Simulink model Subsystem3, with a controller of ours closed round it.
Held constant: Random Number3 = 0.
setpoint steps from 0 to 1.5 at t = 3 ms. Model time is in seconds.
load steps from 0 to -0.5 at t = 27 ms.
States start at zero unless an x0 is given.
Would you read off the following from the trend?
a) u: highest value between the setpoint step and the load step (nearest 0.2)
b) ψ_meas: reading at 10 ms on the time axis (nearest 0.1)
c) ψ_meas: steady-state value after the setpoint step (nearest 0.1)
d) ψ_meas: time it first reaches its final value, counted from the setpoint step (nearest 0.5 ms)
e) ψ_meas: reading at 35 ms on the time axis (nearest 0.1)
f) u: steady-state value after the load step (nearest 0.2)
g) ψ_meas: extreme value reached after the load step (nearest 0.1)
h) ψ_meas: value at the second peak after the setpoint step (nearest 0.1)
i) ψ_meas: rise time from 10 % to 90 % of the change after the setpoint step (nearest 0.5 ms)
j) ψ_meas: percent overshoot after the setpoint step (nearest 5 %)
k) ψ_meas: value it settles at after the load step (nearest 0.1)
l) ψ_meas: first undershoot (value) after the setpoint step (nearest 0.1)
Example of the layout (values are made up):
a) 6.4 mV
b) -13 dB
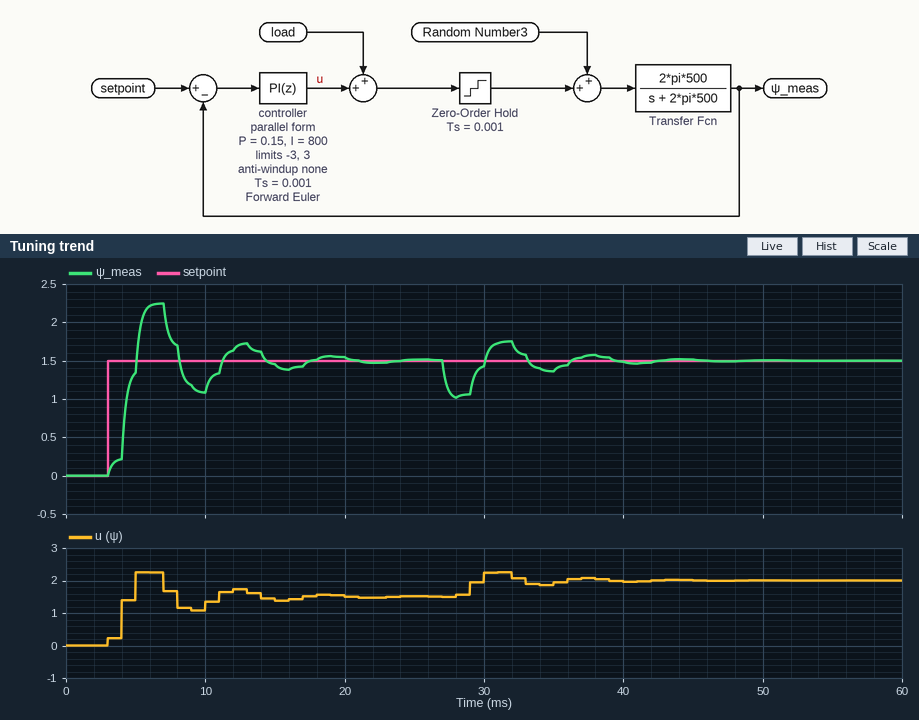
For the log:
a) 2.2
b) 1.1
c) 1.5
d) 2.0 ms
e) 1.4
f) 2.0
g) 1.0
h) 1.7
i) 1.5 ms
j) 50 %
k) 1.5
l) 1.1
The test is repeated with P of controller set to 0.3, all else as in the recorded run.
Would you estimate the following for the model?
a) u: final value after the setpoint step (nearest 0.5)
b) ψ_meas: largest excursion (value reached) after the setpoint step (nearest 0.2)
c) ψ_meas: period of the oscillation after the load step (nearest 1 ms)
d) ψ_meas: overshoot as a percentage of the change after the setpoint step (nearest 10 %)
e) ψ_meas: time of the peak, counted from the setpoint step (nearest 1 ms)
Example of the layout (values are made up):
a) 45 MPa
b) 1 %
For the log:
a) 1.5
b) 2.0
c) 6 ms
d) 40 %
e) 3 ms
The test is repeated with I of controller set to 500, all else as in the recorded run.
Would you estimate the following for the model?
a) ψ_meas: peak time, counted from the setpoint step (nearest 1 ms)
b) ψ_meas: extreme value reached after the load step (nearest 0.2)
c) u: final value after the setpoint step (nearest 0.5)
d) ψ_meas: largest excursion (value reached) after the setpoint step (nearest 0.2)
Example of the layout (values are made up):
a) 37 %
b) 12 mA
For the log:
a) 4 ms
b) 1.0
c) 1.5
d) 1.6
